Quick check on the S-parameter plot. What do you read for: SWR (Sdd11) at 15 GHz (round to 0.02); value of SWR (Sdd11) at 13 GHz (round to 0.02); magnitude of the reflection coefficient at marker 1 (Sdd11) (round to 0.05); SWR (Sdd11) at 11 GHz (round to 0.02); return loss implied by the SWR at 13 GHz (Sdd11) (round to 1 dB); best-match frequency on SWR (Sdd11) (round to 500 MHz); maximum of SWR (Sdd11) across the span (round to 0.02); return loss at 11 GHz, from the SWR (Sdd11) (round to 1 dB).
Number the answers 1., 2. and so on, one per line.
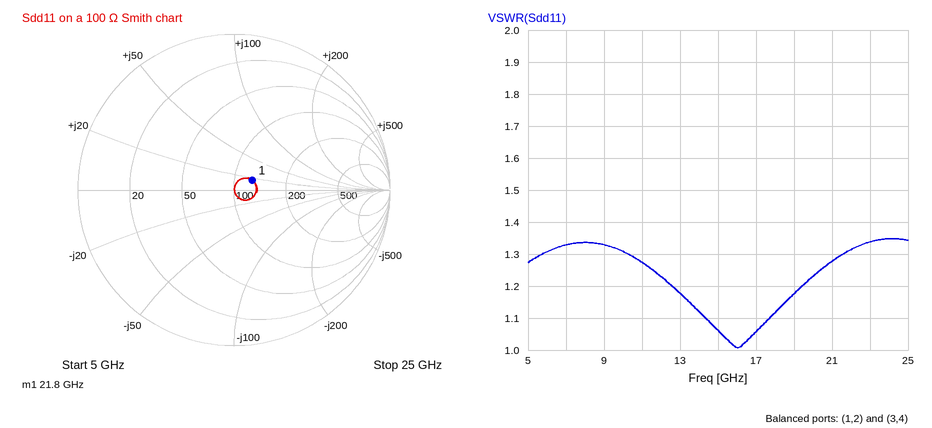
1. 1.06
2. 1.18
3. 0.15
4. 1.28
5. 22 dB
6. 16.0 GHz
7. 1.34
8. 18 dB
